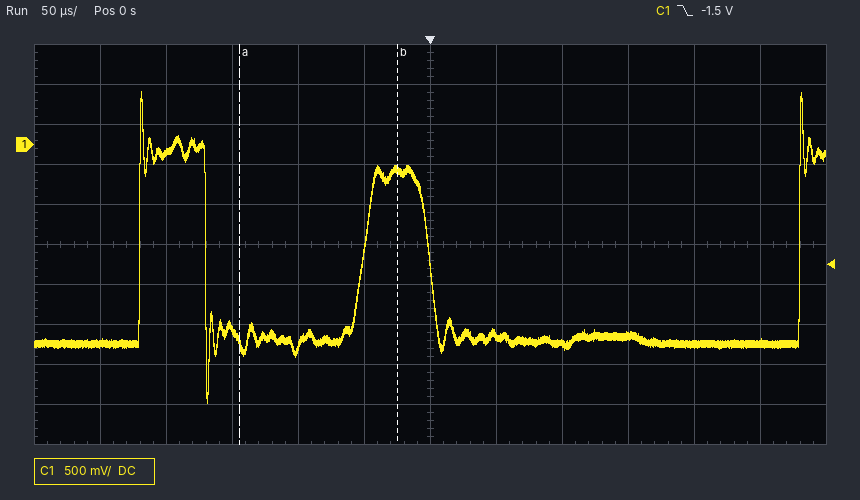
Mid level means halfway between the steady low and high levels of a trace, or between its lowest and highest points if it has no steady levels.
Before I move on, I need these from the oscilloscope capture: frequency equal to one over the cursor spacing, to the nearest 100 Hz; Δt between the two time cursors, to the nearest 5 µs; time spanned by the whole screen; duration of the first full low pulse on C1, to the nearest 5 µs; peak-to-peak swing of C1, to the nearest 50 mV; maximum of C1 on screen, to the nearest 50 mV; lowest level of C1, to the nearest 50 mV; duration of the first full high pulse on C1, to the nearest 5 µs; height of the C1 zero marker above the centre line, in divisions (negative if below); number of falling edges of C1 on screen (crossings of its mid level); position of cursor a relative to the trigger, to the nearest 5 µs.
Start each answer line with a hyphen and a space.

- 8.3 kHz
- 120 µs
- 600 µs
- 120 µs
- 3.90 V
- 650 mV
- -3.25 V
- 50 µs
- +2.5 div
- 2
- -145 µs
